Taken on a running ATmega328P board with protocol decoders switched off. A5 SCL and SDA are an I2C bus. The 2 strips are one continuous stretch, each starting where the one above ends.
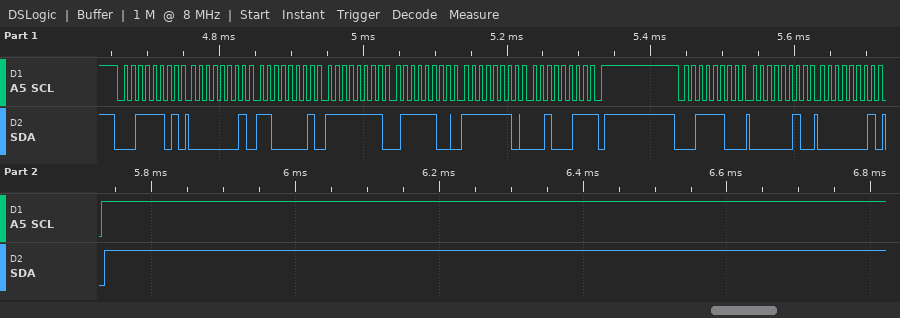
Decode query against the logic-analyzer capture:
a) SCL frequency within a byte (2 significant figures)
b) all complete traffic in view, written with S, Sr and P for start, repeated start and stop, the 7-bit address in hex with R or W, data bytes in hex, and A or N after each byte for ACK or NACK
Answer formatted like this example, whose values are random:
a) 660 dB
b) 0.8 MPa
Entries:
a) 100 kHz
b) S 1ER A 01 A C1 A FF A 7C A FE A 23 N P S 1EW A 02 A 01 A P
